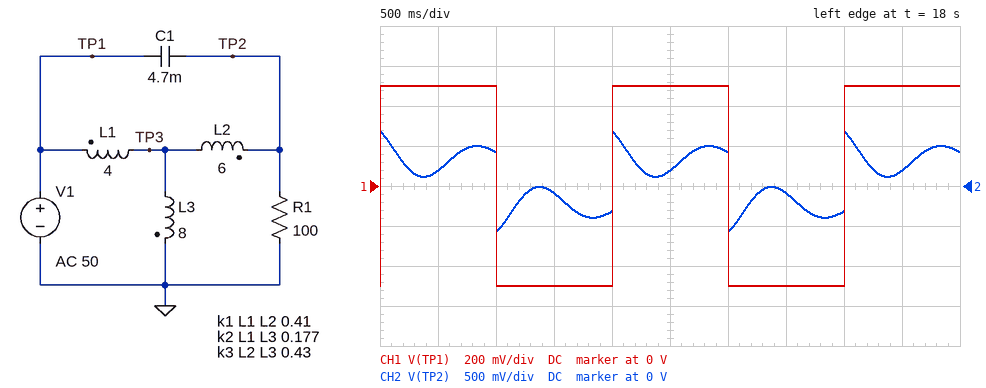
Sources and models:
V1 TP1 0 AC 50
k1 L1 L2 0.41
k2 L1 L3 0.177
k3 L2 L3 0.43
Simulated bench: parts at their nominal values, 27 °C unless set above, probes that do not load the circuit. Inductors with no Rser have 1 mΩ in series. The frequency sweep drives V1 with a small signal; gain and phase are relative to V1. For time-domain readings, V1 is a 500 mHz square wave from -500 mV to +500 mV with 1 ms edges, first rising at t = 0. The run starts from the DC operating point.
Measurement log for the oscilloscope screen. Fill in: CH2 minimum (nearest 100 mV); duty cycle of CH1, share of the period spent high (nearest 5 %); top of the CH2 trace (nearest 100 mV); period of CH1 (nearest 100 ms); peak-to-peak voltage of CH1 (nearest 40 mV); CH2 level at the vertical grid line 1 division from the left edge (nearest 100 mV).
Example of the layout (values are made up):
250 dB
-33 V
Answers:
-600 mV
50 %
700 mV
2.0 s
1.00 V
200 mV
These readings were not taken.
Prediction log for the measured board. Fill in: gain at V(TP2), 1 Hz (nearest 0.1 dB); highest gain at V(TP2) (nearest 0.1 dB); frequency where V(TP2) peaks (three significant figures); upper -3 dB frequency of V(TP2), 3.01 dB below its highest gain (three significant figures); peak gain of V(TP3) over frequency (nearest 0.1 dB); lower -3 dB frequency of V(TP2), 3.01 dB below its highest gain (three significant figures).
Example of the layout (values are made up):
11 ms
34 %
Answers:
-3.8 dB
3.7 dB
1.22 Hz
2.50 Hz
-1.8 dB
1.07 Hz
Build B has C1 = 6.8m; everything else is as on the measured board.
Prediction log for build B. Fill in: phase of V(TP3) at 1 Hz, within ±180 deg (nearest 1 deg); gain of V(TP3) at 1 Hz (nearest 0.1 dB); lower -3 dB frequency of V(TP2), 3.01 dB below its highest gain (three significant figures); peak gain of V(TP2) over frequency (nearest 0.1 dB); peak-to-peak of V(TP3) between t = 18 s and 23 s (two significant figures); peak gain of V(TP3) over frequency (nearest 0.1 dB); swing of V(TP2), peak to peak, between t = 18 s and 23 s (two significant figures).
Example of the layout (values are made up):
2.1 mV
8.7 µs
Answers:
19 deg
-1.8 dB
883 mHz
4.9 dB
790 mV
-1.5 dB
1.1 V
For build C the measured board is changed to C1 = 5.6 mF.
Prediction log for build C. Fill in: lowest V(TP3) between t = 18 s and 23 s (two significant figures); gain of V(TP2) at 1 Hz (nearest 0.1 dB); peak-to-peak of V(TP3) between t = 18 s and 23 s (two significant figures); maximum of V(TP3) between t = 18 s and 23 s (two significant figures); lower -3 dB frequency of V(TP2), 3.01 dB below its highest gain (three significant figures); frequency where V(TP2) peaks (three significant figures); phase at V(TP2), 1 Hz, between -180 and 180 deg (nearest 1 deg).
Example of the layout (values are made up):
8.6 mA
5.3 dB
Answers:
-300 mV
2.5 dB
800 mV
500 mV
975 mHz
1.10 Hz
95 deg
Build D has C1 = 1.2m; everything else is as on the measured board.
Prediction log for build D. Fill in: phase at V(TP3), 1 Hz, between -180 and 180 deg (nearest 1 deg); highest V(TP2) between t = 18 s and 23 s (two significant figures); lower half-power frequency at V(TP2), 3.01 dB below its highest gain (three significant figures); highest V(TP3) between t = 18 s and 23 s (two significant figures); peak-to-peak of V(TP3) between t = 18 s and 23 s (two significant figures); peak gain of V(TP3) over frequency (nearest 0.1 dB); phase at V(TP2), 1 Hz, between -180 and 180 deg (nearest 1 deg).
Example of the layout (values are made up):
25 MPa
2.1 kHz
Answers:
-2 deg
740 mV
2.28 Hz
520 mV
840 mV
-2.2 dB
-19 deg
